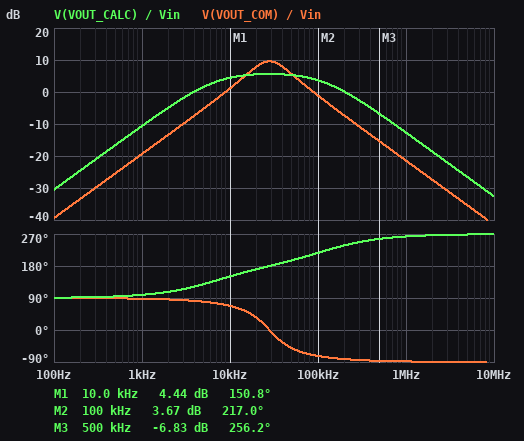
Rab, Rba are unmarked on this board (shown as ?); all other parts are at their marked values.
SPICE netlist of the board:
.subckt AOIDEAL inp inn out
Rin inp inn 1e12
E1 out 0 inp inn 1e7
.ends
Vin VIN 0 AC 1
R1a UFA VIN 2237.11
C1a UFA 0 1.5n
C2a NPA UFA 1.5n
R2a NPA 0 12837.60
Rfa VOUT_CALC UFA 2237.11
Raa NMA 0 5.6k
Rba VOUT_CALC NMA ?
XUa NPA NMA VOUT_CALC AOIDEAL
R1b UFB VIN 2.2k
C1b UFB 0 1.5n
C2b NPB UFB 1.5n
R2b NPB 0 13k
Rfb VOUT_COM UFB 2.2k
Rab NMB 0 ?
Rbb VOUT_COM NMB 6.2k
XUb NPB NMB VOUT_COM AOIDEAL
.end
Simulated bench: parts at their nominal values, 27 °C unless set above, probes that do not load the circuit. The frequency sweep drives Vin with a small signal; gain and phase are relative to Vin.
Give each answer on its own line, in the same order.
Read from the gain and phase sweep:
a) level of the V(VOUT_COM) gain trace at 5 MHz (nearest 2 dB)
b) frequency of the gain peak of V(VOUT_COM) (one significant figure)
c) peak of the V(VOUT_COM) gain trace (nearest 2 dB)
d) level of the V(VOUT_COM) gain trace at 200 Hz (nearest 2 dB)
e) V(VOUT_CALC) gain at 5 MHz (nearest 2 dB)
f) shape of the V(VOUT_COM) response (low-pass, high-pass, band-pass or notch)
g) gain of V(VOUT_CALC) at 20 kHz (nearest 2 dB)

-36 dB
30 kHz
10 dB
-34 dB
-26 dB
band-pass
6 dB
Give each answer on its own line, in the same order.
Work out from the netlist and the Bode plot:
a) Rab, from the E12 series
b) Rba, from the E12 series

8.2 kΩ
22 kΩ
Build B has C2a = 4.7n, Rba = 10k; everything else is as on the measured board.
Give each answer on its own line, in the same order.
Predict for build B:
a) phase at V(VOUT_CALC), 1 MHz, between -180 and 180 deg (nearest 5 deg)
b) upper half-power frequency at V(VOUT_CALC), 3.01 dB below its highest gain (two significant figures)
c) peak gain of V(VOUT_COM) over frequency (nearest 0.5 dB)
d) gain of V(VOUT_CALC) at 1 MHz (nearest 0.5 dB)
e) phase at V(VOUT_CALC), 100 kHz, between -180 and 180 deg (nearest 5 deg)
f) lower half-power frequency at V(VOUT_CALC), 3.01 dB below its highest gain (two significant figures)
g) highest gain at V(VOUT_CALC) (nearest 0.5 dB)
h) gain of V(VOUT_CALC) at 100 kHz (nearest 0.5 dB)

-90 deg
34 kHz
9.5 dB
-17.5 dB
-105 deg
7.4 kHz
14.0 dB
2.5 dB
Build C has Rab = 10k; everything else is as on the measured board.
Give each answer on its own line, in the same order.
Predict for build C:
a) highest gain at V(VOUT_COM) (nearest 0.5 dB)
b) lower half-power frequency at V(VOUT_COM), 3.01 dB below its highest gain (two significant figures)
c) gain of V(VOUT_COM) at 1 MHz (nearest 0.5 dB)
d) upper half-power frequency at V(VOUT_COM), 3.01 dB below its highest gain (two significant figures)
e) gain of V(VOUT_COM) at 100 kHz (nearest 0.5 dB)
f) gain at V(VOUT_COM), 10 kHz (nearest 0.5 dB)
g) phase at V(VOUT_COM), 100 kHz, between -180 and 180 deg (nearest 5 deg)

7.0 dB
16 kHz
-22.0 dB
50 kHz
-2.0 dB
0 dB
-70 deg
